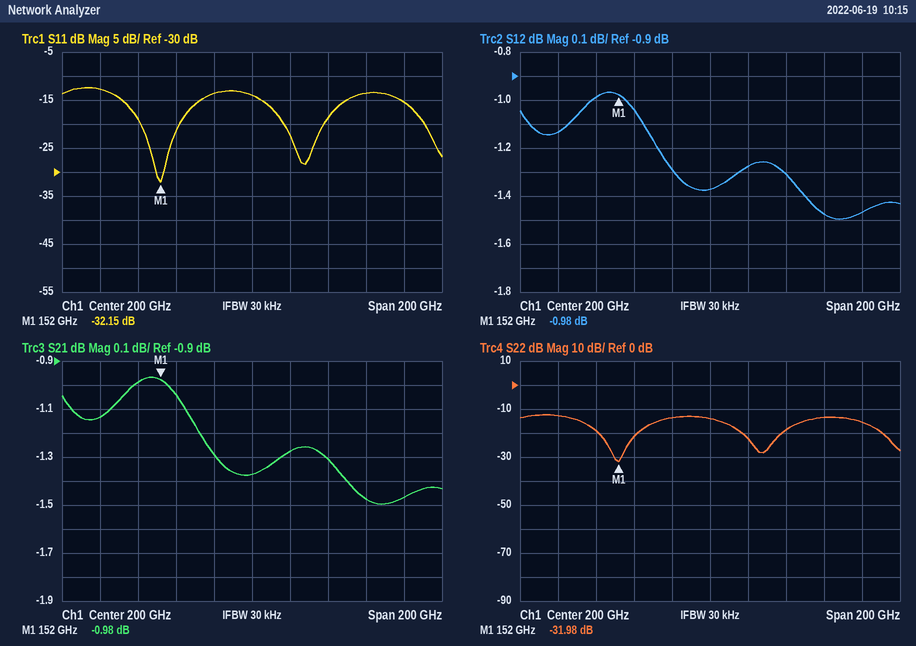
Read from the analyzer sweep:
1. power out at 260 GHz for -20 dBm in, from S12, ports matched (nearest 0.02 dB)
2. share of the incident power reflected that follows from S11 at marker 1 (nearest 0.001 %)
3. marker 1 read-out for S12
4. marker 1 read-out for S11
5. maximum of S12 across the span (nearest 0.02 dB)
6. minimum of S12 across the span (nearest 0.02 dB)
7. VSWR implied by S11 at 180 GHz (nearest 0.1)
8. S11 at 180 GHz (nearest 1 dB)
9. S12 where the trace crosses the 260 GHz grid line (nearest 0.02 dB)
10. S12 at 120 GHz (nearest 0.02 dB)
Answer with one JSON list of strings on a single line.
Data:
["-21.48 dBm", "0.061 %", "-0.98 dB", "-32.15 dB", "-0.96 dB", "-1.50 dB", "1.5", "-14 dB", "-1.48 dB", "-1.14 dB"]
